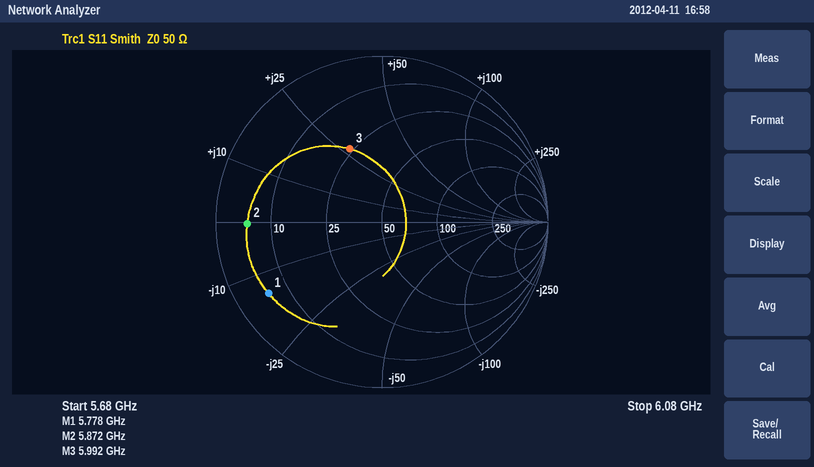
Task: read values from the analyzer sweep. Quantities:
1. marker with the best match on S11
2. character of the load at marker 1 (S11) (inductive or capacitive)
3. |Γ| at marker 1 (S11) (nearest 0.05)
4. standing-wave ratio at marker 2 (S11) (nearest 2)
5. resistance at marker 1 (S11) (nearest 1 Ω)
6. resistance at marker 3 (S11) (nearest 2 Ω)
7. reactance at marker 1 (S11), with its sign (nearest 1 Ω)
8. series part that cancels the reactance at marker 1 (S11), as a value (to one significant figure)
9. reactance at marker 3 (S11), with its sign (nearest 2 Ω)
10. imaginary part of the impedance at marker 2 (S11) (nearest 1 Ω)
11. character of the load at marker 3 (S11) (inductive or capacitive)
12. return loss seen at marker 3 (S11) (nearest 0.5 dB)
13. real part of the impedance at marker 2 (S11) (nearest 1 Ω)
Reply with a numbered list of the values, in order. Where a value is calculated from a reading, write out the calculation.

1. marker 3
2. capacitive
3. 0.80
4. 10
5. 6 Ω
6. 24 Ω
7. -14 Ω
8. L = 14 Ω/(2π × 5.778 GHz) ≈ 386 pH, so 400 pH to one significant figure
9. +28 Ω
10. 0 Ω
11. inductive
12. 6.5 dB
13. 5 Ω
